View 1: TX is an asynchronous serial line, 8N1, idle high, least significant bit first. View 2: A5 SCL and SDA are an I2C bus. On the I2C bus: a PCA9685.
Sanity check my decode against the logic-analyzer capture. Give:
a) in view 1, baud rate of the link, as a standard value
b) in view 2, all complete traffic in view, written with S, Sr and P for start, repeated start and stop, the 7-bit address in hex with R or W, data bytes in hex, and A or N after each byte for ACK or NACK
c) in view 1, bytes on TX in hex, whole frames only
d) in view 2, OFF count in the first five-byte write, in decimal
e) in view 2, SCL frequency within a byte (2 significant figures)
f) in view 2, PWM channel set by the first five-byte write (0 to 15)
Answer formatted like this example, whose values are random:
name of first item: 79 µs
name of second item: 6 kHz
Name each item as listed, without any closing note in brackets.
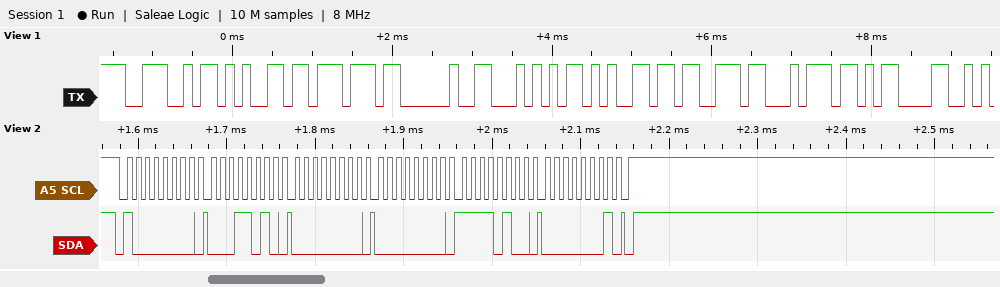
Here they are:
in view 1, baud rate of the link, as a standard value: 9600 baud
in view 2, all complete traffic in view, written with S, Sr and P for start, repeated start and stop, the 7-bit address in hex with R or W, data bytes in hex, and A or N after each byte for ACK or NACK: S 40W A 1A A 00 A 00 A F4 A 01 A P
in view 1, bytes on TX in hex, whole frames only: 4E 65 77 20 54 65 73 74 0D
in view 2, OFF count in the first five-byte write, in decimal: 500
in view 2, SCL frequency within a byte: 100 kHz
in view 2, PWM channel set by the first five-byte write: 5
